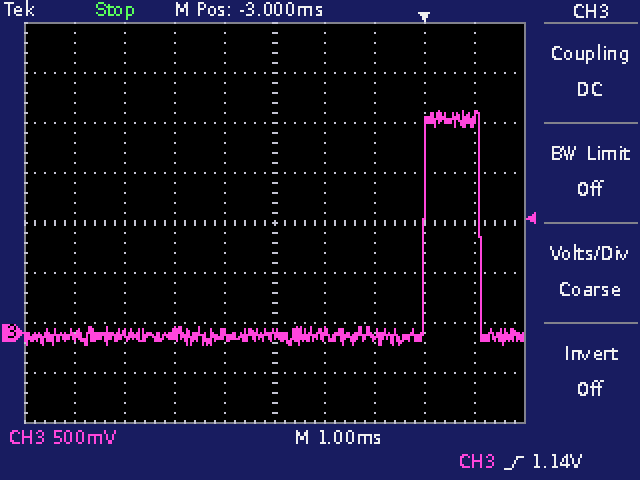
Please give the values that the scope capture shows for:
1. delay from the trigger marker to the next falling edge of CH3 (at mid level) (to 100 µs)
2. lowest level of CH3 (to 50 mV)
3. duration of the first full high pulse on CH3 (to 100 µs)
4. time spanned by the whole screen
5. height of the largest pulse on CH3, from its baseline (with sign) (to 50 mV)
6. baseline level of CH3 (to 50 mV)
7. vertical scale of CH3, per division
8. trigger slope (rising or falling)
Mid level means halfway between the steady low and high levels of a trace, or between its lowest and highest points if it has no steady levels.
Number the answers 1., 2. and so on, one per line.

1. 1.1 ms
2. -100 mV
3. 1.1 ms
4. 10 ms
5. +2.25 V
6. -50 mV
7. 500 mV
8. rising
